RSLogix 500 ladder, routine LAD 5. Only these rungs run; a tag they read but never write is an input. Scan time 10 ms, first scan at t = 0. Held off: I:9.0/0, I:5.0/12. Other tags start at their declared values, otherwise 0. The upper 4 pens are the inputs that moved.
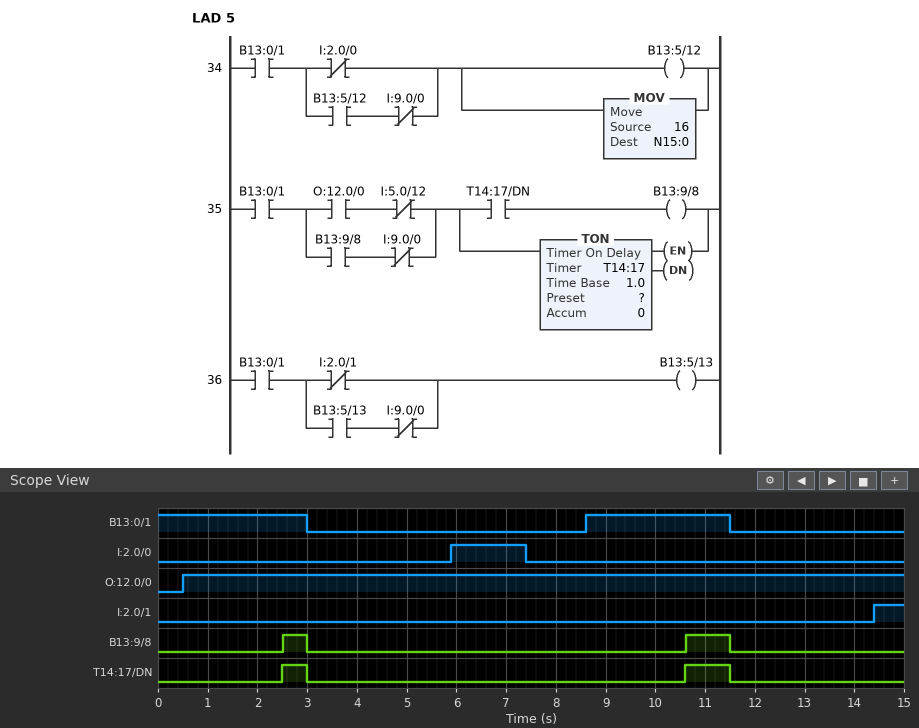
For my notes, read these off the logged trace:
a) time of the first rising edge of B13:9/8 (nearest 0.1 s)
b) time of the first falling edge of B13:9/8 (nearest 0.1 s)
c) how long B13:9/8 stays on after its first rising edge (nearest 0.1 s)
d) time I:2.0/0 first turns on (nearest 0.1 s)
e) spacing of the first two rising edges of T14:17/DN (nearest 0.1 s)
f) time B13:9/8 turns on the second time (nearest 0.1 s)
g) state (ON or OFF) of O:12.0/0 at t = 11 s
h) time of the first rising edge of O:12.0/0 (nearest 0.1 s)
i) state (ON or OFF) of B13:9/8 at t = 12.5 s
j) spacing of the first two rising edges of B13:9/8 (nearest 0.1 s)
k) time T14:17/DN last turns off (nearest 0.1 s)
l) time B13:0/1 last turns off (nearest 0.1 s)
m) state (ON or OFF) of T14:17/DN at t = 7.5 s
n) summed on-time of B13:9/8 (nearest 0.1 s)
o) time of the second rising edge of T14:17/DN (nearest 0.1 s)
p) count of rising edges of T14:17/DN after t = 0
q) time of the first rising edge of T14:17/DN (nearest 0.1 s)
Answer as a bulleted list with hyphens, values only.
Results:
- 2.5 s
- 3.0 s
- 0.5 s
- 5.9 s
- 8.1 s
- 10.6 s
- ON
- 0.5 s
- OFF
- 8.1 s
- 11.5 s
- 11.5 s
- OFF
- 1.4 s
- 10.6 s
- 2
- 2.5 s
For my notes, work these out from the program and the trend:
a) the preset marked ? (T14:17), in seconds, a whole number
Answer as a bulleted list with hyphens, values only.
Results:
- 2 s
